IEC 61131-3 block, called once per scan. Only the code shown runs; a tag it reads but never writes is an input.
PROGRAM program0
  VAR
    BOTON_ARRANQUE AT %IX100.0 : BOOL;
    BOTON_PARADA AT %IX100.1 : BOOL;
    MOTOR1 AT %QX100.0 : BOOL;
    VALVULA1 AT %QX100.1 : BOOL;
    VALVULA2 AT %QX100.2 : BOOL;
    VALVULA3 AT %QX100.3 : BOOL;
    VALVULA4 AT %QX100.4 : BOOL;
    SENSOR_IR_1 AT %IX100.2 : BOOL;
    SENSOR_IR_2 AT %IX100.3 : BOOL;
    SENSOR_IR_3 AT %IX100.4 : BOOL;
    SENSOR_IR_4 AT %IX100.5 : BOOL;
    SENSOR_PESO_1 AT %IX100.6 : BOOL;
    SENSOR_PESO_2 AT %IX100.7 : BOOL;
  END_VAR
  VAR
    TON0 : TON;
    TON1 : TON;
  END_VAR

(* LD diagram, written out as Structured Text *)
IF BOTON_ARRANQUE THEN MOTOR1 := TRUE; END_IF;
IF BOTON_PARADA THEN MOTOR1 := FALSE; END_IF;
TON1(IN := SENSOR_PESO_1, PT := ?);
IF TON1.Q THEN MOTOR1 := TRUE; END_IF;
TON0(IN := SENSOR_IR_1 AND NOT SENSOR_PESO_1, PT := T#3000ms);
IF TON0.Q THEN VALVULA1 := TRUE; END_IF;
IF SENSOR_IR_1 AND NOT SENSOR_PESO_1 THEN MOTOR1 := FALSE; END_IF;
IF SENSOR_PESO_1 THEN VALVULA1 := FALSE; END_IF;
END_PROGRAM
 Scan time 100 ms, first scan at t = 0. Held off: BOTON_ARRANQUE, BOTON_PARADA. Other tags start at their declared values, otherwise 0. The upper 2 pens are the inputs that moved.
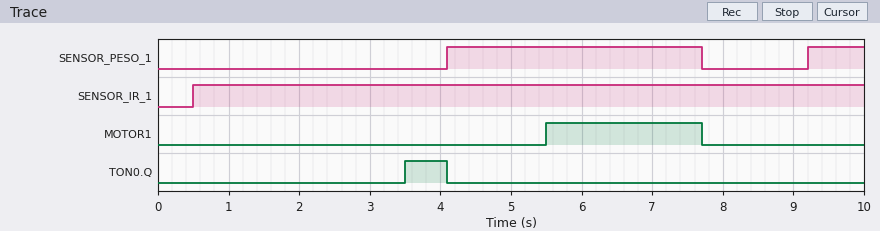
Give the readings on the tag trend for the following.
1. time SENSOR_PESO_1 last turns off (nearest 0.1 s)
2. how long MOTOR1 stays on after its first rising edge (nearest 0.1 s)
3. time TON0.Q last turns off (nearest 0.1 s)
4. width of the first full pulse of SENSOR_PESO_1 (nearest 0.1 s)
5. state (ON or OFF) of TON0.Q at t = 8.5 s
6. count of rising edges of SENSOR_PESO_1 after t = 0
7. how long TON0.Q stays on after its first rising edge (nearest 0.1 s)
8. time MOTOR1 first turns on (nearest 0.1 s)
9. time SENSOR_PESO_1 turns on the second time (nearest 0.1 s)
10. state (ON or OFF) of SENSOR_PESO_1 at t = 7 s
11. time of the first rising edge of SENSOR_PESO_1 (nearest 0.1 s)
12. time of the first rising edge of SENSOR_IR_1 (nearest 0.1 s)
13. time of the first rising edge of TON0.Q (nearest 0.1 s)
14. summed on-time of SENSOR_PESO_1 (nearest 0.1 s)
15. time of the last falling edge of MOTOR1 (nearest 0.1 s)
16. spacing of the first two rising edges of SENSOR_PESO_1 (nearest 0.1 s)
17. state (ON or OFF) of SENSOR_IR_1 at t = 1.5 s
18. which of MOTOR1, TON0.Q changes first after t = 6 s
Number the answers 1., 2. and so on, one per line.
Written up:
1. 7.7 s
2. 2.2 s
3. 4.1 s
4. 3.6 s
5. OFF
6. 2
7. 0.6 s
8. 5.5 s
9. 9.2 s
10. ON
11. 4.1 s
12. 0.5 s
13. 3.5 s
14. 4.4 s
15. 7.7 s
16. 5.1 s
17. ON
18. MOTOR1
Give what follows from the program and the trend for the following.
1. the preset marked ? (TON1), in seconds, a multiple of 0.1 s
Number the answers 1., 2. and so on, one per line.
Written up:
1. 1.4 s
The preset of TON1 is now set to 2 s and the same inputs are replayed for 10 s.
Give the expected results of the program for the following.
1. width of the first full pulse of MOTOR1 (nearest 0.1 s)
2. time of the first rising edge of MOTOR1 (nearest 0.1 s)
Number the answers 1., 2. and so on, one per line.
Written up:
1. 1.6 s
2. 6.1 s
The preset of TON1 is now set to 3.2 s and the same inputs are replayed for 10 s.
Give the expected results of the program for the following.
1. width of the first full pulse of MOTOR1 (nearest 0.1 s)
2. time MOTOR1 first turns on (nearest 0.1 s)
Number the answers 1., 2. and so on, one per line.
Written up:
1. 0.4 s
2. 7.3 s
